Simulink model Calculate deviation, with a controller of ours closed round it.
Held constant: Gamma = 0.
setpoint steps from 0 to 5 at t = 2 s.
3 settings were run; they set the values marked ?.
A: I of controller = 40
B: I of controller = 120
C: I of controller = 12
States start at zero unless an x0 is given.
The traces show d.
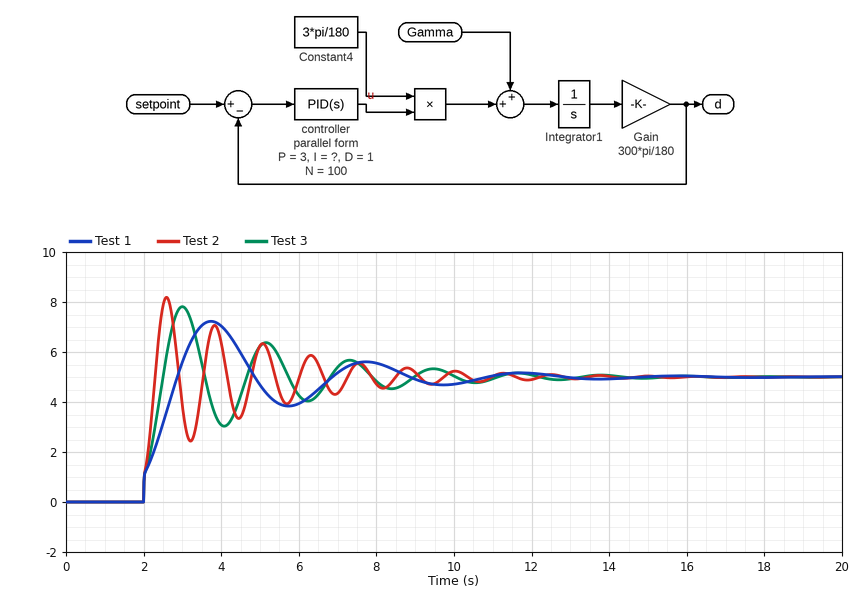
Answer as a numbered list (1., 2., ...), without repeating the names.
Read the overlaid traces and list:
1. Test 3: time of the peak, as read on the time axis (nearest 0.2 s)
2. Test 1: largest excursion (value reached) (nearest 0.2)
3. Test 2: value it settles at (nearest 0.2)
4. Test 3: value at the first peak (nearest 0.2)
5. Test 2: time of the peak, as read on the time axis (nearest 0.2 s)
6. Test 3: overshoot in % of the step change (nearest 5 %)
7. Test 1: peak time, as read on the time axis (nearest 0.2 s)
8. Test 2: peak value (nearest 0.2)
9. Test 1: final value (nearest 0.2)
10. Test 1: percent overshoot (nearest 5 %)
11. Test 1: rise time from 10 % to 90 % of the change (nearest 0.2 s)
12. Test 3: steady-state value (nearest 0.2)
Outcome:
1. 3.0 s
2. 7.2
3. 5.0
4. 7.8
5. 2.6 s
6. 55 %
7. 3.8 s
8. 8.2
9. 5.0
10. 45 %
11. 0.8 s
12. 5.0
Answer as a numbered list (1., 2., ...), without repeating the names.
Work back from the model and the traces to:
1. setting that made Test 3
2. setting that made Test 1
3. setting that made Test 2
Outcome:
1. A
2. C
3. B
